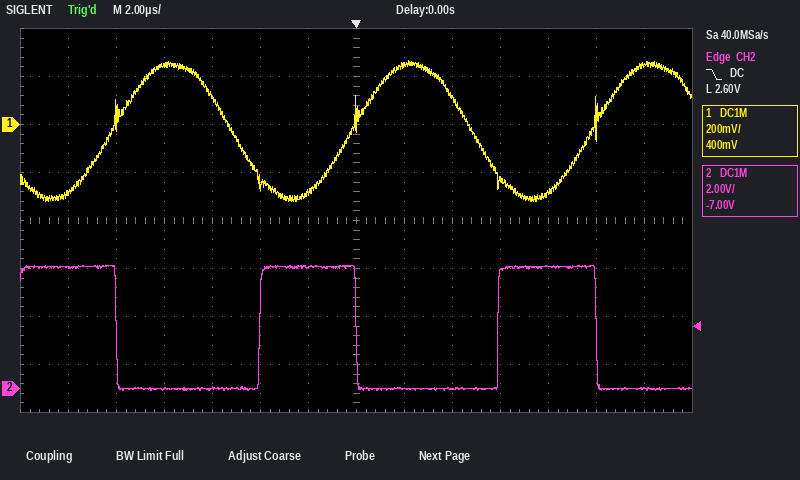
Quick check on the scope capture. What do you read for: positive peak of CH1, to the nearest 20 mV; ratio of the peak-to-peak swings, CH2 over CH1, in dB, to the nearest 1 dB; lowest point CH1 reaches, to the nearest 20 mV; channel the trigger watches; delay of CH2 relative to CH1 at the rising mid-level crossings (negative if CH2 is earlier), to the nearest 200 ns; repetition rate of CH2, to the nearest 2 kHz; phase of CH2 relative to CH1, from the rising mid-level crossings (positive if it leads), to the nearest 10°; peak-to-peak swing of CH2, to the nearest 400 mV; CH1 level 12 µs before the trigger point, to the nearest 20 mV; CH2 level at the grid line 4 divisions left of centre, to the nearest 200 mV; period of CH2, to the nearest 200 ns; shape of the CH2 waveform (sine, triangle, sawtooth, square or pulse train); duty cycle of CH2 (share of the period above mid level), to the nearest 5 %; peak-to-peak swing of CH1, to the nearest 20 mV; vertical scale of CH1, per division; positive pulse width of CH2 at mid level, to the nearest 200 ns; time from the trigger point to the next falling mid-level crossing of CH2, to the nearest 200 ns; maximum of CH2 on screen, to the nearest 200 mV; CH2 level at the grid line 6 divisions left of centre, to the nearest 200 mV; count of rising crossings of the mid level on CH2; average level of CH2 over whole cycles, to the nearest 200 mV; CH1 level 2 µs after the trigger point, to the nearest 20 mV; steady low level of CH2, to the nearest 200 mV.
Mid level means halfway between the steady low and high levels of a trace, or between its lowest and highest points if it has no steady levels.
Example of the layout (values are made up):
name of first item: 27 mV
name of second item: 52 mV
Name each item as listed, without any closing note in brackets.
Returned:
positive peak of CH1, to the nearest 20 mV: 260 mV
ratio of the peak-to-peak swings, CH2 over CH1, in dB, to the nearest 1 dB: 19 dB
lowest point CH1 reaches, to the nearest 20 mV: -320 mV
channel the trigger watches: CH2
delay of CH2 relative to CH1 at the rising mid-level crossings (negative if CH2 is earlier), to the nearest 200 ns: -3.8 µs
repetition rate of CH2, to the nearest 2 kHz: 100 kHz
phase of CH2 relative to CH1, from the rising mid-level crossings (positive if it leads), to the nearest 10°: +140°
peak-to-peak swing of CH2, to the nearest 400 mV: 5.2 V
CH1 level 12 µs before the trigger point, to the nearest 20 mV: -280 mV
CH2 level at the grid line 4 divisions left of centre, to the nearest 200 mV: 0.0 V
period of CH2, to the nearest 200 ns: 10.0 µs
shape of the CH2 waveform: pulse train
duty cycle of CH2 (share of the period above mid level), to the nearest 5 %: 40 %
peak-to-peak swing of CH1, to the nearest 20 mV: 580 mV
vertical scale of CH1, per division: 200 mV
positive pulse width of CH2 at mid level, to the nearest 200 ns: 4.0 µs
time from the trigger point to the next falling mid-level crossing of CH2, to the nearest 200 ns: 10.0 µs
maximum of CH2 on screen, to the nearest 200 mV: 5.2 V
CH2 level at the grid line 6 divisions left of centre, to the nearest 200 mV: 5.0 V
count of rising crossings of the mid level on CH2: 2
average level of CH2 over whole cycles, to the nearest 200 mV: 2.0 V
CH1 level 2 µs after the trigger point, to the nearest 20 mV: 240 mV
steady low level of CH2, to the nearest 200 mV: 0.0 V
